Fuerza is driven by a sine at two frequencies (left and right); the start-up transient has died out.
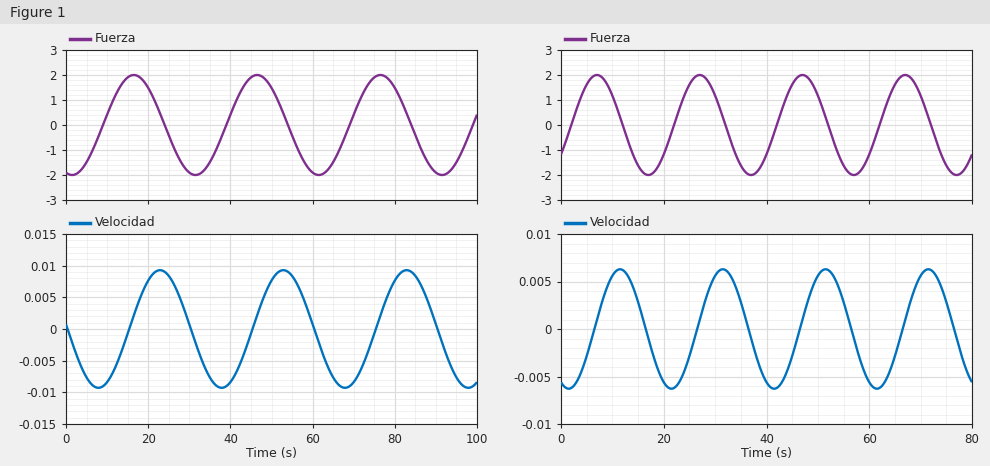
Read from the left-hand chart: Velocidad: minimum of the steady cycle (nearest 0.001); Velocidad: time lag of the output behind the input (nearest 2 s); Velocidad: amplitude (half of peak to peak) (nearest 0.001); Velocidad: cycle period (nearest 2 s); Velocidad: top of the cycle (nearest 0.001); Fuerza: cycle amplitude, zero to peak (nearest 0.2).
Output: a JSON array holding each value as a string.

["-0.009", "6 s", "0.009", "30 s", "0.009", "2.0"]
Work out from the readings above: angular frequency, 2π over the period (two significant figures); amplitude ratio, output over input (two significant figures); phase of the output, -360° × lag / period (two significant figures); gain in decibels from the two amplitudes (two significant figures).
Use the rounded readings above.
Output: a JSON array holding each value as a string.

["0.21 rad/s", "0.0045", "-72°", "-47 dB"]
